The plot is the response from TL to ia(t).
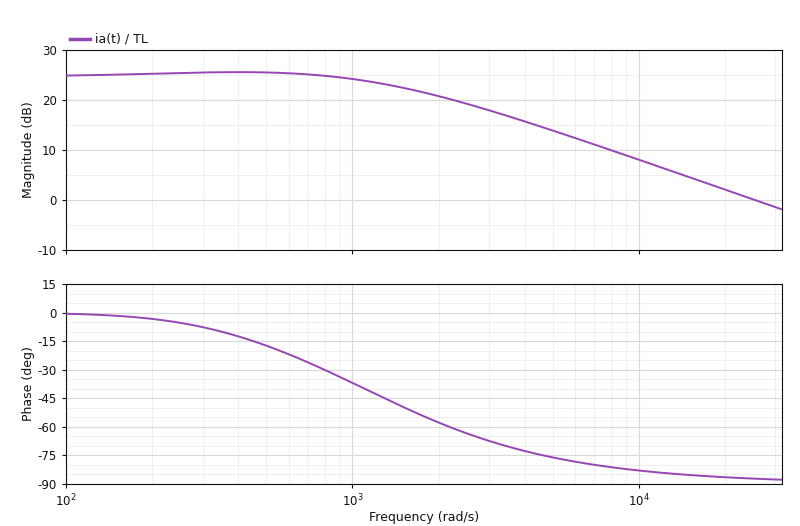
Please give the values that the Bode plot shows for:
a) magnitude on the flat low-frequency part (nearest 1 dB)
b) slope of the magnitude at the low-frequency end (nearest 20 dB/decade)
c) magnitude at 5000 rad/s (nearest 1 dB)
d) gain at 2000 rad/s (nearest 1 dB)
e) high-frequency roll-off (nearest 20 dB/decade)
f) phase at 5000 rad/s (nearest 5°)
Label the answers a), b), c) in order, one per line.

a) 25 dB
b) 0 dB/decade
c) 14 dB
d) 21 dB
e) -20 dB/decade
f) -75°
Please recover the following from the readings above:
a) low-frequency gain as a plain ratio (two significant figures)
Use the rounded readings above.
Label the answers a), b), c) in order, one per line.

a) 18
